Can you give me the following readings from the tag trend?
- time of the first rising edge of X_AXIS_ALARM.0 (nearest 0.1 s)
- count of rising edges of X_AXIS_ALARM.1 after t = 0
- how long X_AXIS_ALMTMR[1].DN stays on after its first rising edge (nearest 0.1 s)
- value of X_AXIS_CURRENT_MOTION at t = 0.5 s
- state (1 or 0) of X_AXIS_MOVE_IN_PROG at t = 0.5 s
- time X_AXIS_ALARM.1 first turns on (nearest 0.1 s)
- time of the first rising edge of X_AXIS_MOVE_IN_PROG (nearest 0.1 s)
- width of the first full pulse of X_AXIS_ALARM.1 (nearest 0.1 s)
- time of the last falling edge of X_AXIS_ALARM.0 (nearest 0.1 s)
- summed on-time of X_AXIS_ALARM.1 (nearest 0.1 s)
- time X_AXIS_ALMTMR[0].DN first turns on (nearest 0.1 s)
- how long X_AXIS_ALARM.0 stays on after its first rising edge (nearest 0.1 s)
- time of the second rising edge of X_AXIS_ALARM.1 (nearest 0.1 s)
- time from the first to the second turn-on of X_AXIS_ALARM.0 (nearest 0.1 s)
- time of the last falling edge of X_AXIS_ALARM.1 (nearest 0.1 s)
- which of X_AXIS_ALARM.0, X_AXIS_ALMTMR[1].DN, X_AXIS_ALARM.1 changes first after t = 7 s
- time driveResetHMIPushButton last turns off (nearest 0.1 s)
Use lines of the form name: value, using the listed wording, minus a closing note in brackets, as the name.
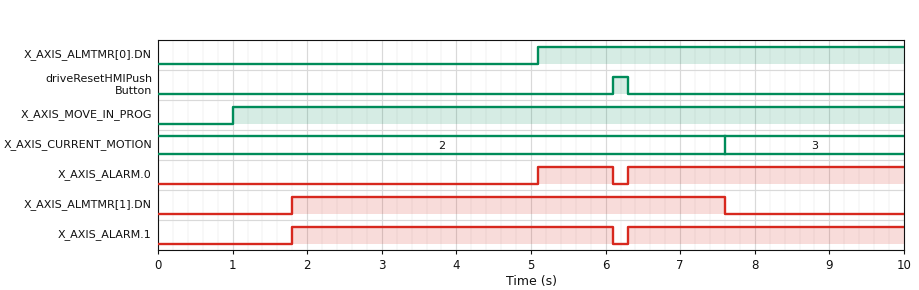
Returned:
time of the first rising edge of X_AXIS_ALARM.0: 5.1 s
count of rising edges of X_AXIS_ALARM.1 after t = 0: 2
how long X_AXIS_ALMTMR[1].DN stays on after its first rising edge: 5.8 s
value of X_AXIS_CURRENT_MOTION at t = 0.5 s: 2
state (1 or 0) of X_AXIS_MOVE_IN_PROG at t = 0.5 s: 0
time X_AXIS_ALARM.1 first turns on: 1.8 s
time of the first rising edge of X_AXIS_MOVE_IN_PROG: 1.0 s
width of the first full pulse of X_AXIS_ALARM.1: 4.3 s
time of the last falling edge of X_AXIS_ALARM.0: 6.1 s
summed on-time of X_AXIS_ALARM.1: 8.0 s
time X_AXIS_ALMTMR[0].DN first turns on: 5.1 s
how long X_AXIS_ALARM.0 stays on after its first rising edge: 1.0 s
time of the second rising edge of X_AXIS_ALARM.1: 6.3 s
time from the first to the second turn-on of X_AXIS_ALARM.0: 1.2 s
time of the last falling edge of X_AXIS_ALARM.1: 6.1 s
which of X_AXIS_ALARM.0, X_AXIS_ALMTMR[1].DN, X_AXIS_ALARM.1 changes first after t = 7 s: X_AXIS_ALMTMR[1].DN
time driveResetHMIPushButton last turns off: 6.3 s
